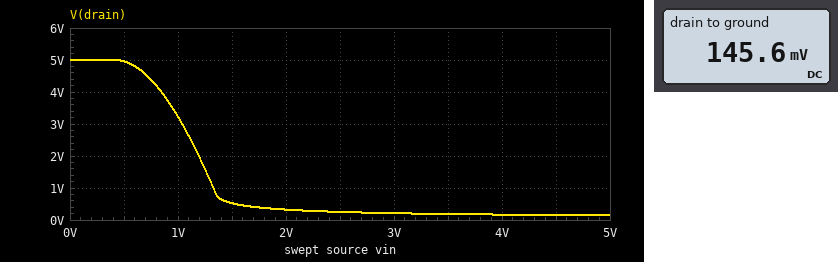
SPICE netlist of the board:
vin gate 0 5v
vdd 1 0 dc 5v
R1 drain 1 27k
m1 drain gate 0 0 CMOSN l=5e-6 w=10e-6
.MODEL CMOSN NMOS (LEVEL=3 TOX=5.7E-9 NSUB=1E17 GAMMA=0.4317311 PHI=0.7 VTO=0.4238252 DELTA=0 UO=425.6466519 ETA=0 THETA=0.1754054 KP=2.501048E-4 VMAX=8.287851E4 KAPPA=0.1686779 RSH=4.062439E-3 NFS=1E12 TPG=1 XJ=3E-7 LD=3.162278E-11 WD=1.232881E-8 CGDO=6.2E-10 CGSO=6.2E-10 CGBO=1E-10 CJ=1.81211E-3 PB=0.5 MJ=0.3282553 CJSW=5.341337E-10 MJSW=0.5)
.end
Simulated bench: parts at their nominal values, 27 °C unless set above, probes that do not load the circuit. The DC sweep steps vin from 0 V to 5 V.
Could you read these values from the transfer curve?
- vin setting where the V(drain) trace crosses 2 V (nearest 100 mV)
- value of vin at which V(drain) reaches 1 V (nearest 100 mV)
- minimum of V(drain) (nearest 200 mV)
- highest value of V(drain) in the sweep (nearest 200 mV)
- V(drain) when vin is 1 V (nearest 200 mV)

1.2 V
1.3 V
200 mV
5.0 V
3.2 V
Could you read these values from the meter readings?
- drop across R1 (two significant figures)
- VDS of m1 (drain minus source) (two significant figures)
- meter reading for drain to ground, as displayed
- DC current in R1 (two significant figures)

4.9 V
150 mV
145.6 mV
180 µA
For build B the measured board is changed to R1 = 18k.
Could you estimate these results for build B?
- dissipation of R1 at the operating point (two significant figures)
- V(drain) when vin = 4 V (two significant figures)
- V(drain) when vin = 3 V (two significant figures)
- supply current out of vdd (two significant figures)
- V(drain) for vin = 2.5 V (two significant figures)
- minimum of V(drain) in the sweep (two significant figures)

1.3 mW
250 mV
320 mV
270 µA
390 mV
220 mV
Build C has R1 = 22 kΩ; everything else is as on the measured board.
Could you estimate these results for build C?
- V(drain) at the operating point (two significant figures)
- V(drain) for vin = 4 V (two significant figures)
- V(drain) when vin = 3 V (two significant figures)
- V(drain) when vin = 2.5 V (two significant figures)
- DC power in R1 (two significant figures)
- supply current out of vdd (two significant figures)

180 mV
210 mV
260 mV
310 mV
1.1 mW
220 µA
